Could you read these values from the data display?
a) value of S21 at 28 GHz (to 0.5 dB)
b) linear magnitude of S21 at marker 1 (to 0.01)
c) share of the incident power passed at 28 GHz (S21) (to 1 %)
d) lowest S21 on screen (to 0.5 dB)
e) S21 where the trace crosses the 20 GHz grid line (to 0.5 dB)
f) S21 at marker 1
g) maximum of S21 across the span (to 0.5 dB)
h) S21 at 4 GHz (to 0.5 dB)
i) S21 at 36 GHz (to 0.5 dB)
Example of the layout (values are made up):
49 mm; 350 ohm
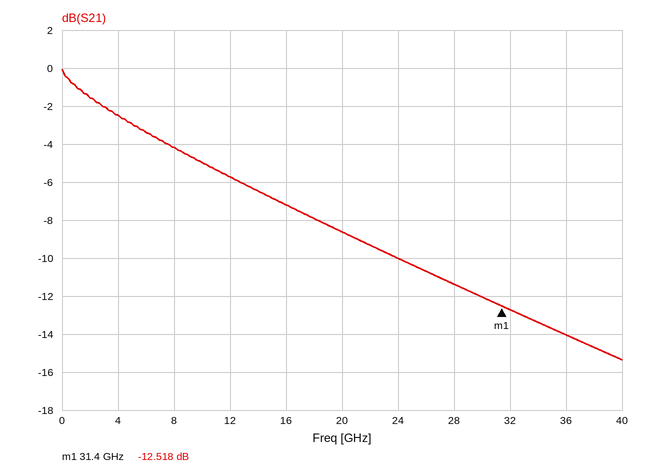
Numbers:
-11.5 dB; 0.24; 7 %; -15.5 dB; -8.5 dB; -12.518 dB; 0.0 dB; -2.5 dB; -14.0 dB
